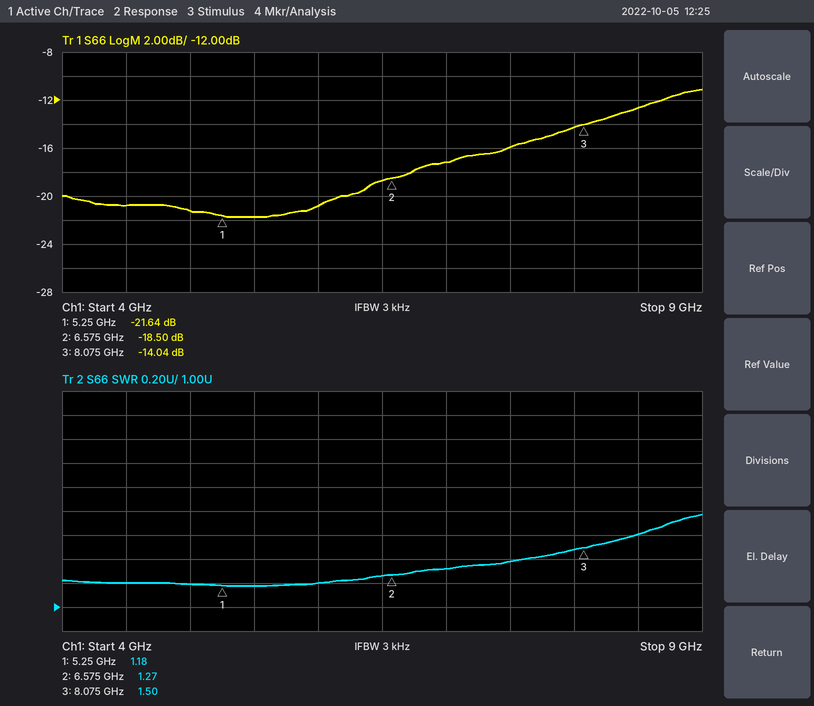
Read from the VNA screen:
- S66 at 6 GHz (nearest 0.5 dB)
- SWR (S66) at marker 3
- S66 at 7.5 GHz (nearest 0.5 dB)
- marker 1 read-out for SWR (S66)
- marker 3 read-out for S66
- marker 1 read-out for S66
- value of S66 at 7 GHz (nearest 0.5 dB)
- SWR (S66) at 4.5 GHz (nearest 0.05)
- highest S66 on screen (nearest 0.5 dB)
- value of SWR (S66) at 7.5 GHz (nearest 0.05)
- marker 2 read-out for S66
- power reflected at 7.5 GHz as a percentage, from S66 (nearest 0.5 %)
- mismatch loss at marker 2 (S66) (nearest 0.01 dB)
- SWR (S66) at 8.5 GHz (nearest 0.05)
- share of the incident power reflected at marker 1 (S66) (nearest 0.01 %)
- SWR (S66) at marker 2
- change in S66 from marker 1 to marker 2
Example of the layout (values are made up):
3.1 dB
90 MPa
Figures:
-21.0 dB
1.50
-16.0 dB
1.18
-14.04 dB
-21.64 dB
-17.0 dB
1.20
-11.0 dB
1.40
-18.50 dB
2.5 %
0.06 dB
1.60
0.69 %
1.27
3.14 dB
